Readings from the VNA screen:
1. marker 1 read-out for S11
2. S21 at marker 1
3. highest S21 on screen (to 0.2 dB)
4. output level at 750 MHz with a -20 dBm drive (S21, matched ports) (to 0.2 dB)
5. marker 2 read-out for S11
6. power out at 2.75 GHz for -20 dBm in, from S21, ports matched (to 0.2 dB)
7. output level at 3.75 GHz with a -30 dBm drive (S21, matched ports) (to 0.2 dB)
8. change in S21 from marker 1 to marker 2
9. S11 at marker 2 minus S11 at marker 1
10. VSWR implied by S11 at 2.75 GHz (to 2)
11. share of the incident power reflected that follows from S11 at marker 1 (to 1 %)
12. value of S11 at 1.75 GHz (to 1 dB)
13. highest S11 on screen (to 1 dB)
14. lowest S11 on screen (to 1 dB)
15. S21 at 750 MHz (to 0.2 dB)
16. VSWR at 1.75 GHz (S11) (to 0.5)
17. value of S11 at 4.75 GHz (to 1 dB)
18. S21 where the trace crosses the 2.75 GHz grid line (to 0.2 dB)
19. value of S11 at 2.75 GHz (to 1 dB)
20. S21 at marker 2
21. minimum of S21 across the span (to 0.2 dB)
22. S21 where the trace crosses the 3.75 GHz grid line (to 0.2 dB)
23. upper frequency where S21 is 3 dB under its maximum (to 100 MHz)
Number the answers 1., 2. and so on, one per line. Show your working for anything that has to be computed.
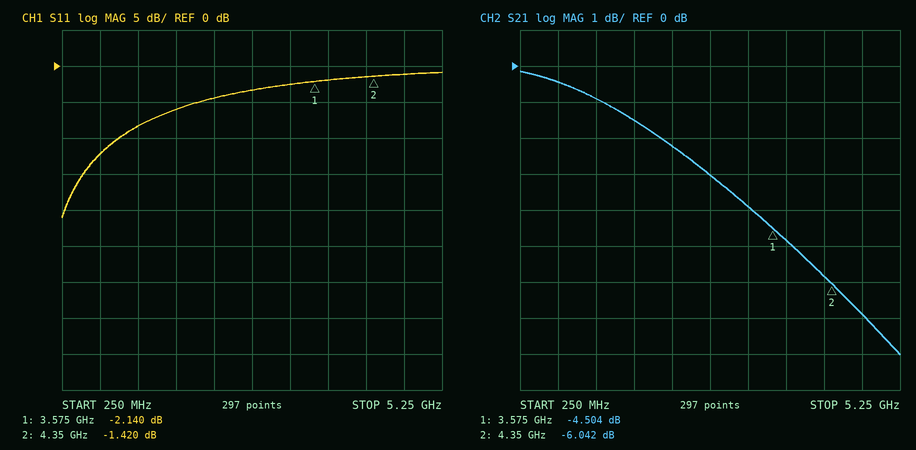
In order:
1. -2.140 dB
2. -4.504 dB
3. -0.2 dB
4. -20 dBm + (-0.4 dB) = -20.4 dBm
5. -1.420 dB
6. -20 dBm + (-3.0 dB) = -23.0 dBm
7. -30 dBm + (-4.8 dB) = -34.8 dBm
8. -6.042 − (-4.504) = -1.538 dB
9. -1.42 − (-2.14) = 0.720 dB
10. |Γ| = 10^(-3/20) = 0.7079; VSWR = (1 + 0.7079)/(1 − 0.7079) ≈ 6
11. 10^(-2.14/10) ≈ 61 %
12. -6 dB
13. -1 dB
14. -21 dB
15. -0.4 dB
16. |Γ| = 10^(-6/20) = 0.5012; VSWR = (1 + 0.5012)/(1 − 0.5012) ≈ 3.0
17. -1 dB
18. -3.0 dB
19. -3 dB
20. -6.042 dB
21. -8.0 dB
22. -4.8 dB
23. 2.8 GHz
